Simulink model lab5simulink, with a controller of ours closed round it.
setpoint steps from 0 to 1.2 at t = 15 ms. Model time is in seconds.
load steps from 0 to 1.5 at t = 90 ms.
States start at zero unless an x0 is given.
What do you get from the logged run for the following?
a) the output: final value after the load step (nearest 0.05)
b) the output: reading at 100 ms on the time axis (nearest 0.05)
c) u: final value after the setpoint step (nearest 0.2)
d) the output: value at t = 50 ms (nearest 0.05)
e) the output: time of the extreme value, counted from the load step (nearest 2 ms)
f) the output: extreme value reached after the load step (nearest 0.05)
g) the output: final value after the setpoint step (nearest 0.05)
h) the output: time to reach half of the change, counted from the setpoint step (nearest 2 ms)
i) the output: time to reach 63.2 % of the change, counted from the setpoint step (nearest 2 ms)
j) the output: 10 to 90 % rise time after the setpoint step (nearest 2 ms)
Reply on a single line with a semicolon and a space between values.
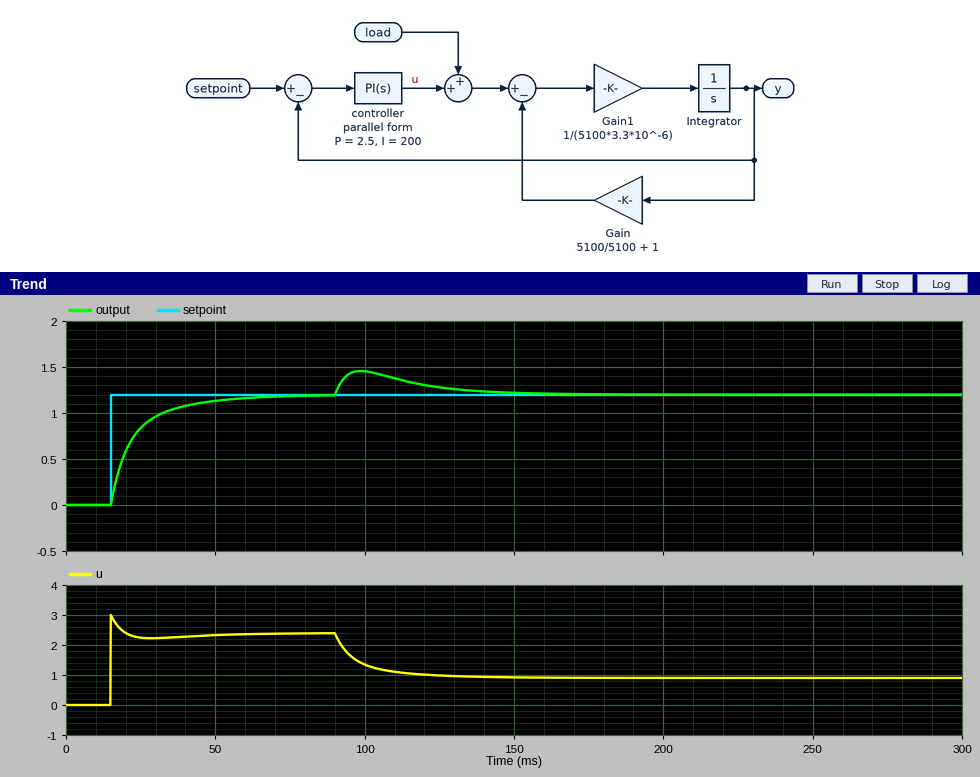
1.20; 1.45; 2.4; 1.15; 8 ms; 1.45; 1.20; 6 ms; 8 ms; 24 ms
